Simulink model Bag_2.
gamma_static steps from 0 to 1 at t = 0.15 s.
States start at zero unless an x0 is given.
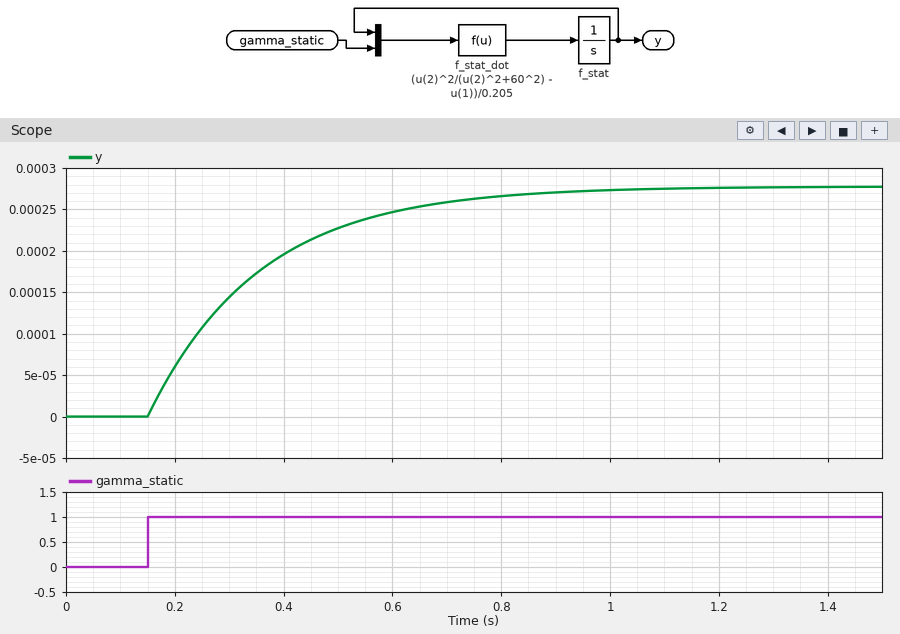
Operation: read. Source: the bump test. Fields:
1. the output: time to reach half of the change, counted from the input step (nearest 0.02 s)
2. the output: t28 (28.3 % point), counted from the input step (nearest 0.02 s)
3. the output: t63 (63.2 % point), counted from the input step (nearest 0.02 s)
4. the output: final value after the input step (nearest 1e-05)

0.14 s
0.06 s
0.20 s
0.00028
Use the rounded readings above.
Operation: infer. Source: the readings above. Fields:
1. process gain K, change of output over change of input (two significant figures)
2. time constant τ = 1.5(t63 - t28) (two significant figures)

0.00028
0.21 s
